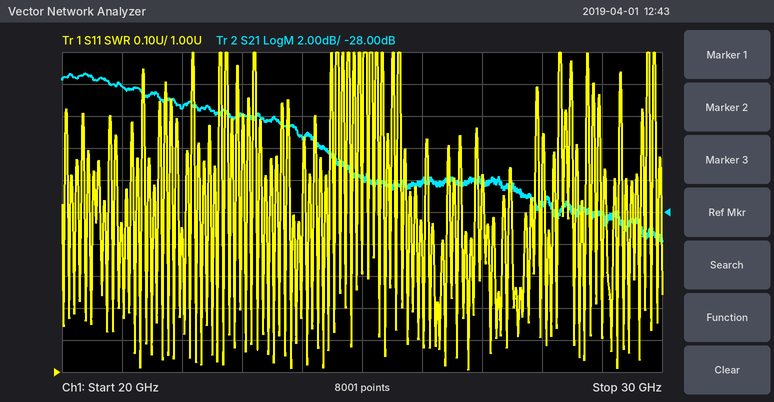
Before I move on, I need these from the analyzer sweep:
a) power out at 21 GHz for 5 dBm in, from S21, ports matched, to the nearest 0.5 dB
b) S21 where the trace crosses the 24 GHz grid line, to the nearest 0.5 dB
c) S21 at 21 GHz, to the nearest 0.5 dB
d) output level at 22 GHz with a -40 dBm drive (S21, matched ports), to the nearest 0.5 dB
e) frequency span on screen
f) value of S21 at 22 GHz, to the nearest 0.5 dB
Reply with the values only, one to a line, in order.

-15.0 dBm
-23.5 dB
-20.0 dB
-61.5 dBm
10 GHz
-21.5 dB
